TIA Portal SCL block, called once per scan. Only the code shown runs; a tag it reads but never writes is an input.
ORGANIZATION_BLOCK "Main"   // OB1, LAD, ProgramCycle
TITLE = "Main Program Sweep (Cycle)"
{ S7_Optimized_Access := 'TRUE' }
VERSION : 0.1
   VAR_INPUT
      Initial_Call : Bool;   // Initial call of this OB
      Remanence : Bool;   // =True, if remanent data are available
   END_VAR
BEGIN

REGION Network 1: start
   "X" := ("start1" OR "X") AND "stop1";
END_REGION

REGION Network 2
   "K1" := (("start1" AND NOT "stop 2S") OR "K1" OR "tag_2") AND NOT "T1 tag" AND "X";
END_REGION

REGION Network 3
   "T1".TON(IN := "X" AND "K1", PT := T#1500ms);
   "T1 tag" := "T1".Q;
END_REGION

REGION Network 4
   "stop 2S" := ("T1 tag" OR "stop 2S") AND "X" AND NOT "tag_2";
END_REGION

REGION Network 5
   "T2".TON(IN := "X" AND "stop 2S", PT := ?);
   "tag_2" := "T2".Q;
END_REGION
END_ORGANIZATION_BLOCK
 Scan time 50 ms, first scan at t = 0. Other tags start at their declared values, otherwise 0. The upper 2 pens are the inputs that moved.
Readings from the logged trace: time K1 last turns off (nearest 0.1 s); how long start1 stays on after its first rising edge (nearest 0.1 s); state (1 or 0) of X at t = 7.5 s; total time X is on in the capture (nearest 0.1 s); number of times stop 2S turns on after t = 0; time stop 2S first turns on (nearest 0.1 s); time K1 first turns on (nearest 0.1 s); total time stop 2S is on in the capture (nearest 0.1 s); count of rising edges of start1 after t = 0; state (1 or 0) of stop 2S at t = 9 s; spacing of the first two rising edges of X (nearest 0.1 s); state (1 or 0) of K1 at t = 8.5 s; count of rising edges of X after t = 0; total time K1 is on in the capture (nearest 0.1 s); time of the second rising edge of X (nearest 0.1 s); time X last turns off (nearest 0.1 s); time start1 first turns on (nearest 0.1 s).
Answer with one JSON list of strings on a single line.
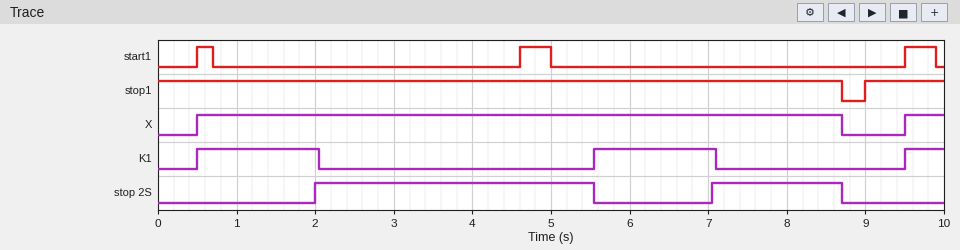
["7.1 s", "0.2 s", "1", "8.7 s", "2", "2.0 s", "0.5 s", "5.2 s", "3", "0", "9.0 s", "0", "2", "3.6 s", "9.5 s", "8.7 s", "0.5 s"]
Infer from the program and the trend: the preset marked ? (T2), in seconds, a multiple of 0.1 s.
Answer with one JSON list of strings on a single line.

["3.5 s"]
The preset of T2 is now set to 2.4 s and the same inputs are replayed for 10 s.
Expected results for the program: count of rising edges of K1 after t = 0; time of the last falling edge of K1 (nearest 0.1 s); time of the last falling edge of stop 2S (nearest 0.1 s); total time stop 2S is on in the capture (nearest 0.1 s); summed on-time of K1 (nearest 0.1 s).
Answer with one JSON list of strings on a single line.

["4", "8.7 s", "8.4 s", "4.9 s", "3.9 s"]
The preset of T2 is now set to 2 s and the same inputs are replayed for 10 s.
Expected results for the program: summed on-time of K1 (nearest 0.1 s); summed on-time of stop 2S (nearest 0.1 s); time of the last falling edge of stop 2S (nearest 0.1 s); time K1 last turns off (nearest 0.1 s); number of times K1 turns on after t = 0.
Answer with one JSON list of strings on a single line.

["4.7 s", "4.1 s", "7.6 s", "8.7 s", "4"]
